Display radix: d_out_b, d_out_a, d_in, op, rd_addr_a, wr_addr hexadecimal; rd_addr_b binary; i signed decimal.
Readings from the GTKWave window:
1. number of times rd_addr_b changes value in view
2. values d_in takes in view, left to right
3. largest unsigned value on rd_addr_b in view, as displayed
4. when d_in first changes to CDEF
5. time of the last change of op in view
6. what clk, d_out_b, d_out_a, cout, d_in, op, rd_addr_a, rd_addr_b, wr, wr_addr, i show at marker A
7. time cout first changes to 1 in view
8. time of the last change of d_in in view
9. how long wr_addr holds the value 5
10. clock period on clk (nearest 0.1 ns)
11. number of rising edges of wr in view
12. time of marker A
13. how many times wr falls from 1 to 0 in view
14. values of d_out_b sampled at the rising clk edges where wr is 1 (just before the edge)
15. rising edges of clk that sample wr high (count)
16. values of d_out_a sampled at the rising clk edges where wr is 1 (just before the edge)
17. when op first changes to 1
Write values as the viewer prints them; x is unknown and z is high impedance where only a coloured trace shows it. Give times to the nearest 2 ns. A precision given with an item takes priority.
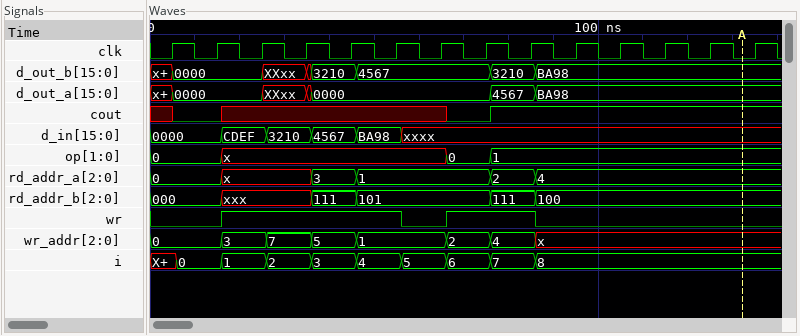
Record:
5
0000, CDEF, 3210, 4567, BA98, xxxx
111
16 ns
76 ns
clk=0, d_out_b=BA98, d_out_a=BA98, cout=1, d_in=xxxx, op=1, rd_addr_a=4, rd_addr_b=100, wr=0, wr_addr=x, i=8
76 ns
56 ns
10 ns
10 ns
2
132 ns
2
0000, XXxx, 3210, 4567, 4567, 3210
6
0000, XXxx, 0000, 0000, 0000, 4567
76 ns
